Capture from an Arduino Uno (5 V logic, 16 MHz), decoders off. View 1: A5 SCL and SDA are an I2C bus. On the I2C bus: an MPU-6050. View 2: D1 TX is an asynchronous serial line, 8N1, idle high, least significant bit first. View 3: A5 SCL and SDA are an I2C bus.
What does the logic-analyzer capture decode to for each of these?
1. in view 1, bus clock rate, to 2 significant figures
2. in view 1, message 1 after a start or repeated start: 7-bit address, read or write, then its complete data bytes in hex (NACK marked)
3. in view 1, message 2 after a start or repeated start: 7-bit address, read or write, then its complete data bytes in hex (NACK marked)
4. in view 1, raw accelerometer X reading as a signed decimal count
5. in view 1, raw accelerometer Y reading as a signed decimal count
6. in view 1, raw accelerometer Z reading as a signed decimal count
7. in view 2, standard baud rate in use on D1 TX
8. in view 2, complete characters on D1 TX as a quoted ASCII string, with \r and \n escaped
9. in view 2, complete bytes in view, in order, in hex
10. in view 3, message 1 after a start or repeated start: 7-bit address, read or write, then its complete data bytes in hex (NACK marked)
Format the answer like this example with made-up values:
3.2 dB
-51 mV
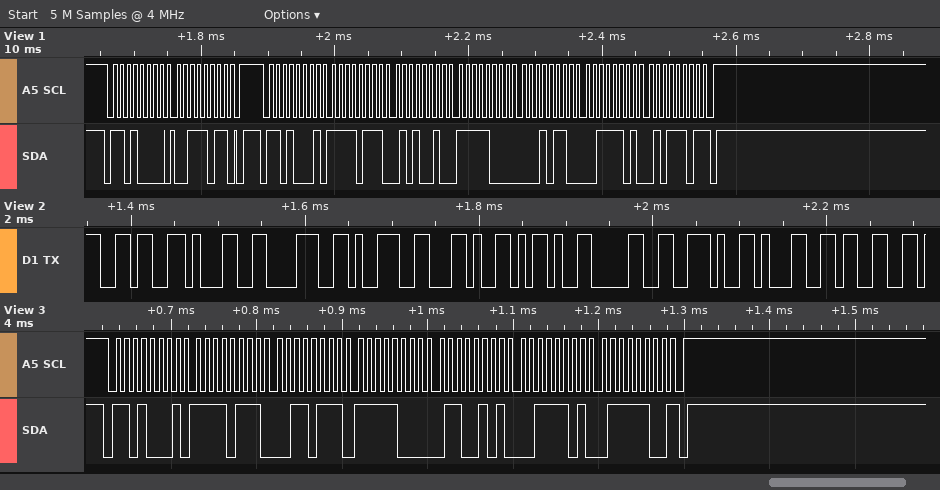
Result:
100 kHz
0x68 write: 3B
0x68 read: F7 52 F8 16 3D 5D NACK
-2222
-2026
15709
115200 baud
"6189,-0.13"
0x36 0x31 0x38 0x39 0x2C 0x2D 0x30 0x2E 0x31 0x33
0x68 read: F7 37 F8 65 3D 7C NACK
